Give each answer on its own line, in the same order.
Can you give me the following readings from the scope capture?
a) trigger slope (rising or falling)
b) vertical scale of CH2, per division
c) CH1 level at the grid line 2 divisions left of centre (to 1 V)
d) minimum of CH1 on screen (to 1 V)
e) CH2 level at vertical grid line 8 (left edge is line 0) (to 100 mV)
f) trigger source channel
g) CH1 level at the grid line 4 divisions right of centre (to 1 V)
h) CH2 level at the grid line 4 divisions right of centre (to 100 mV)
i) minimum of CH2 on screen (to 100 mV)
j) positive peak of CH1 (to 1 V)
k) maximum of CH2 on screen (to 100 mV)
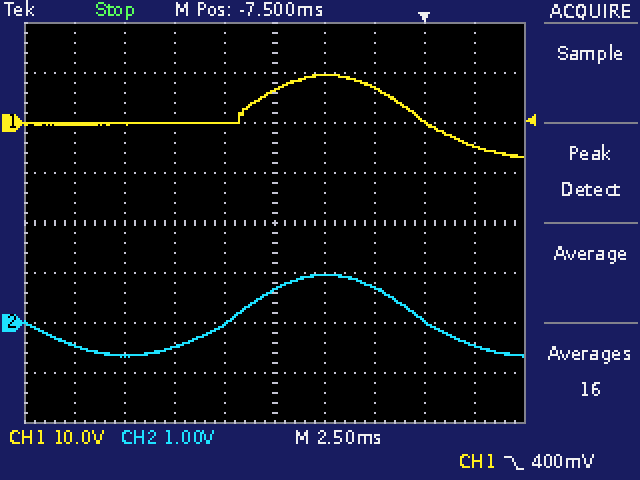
falling
1 V
0 V
-7 V
0.0 V
CH1
-5 V
-500 mV
-700 mV
10 V
1.0 V
